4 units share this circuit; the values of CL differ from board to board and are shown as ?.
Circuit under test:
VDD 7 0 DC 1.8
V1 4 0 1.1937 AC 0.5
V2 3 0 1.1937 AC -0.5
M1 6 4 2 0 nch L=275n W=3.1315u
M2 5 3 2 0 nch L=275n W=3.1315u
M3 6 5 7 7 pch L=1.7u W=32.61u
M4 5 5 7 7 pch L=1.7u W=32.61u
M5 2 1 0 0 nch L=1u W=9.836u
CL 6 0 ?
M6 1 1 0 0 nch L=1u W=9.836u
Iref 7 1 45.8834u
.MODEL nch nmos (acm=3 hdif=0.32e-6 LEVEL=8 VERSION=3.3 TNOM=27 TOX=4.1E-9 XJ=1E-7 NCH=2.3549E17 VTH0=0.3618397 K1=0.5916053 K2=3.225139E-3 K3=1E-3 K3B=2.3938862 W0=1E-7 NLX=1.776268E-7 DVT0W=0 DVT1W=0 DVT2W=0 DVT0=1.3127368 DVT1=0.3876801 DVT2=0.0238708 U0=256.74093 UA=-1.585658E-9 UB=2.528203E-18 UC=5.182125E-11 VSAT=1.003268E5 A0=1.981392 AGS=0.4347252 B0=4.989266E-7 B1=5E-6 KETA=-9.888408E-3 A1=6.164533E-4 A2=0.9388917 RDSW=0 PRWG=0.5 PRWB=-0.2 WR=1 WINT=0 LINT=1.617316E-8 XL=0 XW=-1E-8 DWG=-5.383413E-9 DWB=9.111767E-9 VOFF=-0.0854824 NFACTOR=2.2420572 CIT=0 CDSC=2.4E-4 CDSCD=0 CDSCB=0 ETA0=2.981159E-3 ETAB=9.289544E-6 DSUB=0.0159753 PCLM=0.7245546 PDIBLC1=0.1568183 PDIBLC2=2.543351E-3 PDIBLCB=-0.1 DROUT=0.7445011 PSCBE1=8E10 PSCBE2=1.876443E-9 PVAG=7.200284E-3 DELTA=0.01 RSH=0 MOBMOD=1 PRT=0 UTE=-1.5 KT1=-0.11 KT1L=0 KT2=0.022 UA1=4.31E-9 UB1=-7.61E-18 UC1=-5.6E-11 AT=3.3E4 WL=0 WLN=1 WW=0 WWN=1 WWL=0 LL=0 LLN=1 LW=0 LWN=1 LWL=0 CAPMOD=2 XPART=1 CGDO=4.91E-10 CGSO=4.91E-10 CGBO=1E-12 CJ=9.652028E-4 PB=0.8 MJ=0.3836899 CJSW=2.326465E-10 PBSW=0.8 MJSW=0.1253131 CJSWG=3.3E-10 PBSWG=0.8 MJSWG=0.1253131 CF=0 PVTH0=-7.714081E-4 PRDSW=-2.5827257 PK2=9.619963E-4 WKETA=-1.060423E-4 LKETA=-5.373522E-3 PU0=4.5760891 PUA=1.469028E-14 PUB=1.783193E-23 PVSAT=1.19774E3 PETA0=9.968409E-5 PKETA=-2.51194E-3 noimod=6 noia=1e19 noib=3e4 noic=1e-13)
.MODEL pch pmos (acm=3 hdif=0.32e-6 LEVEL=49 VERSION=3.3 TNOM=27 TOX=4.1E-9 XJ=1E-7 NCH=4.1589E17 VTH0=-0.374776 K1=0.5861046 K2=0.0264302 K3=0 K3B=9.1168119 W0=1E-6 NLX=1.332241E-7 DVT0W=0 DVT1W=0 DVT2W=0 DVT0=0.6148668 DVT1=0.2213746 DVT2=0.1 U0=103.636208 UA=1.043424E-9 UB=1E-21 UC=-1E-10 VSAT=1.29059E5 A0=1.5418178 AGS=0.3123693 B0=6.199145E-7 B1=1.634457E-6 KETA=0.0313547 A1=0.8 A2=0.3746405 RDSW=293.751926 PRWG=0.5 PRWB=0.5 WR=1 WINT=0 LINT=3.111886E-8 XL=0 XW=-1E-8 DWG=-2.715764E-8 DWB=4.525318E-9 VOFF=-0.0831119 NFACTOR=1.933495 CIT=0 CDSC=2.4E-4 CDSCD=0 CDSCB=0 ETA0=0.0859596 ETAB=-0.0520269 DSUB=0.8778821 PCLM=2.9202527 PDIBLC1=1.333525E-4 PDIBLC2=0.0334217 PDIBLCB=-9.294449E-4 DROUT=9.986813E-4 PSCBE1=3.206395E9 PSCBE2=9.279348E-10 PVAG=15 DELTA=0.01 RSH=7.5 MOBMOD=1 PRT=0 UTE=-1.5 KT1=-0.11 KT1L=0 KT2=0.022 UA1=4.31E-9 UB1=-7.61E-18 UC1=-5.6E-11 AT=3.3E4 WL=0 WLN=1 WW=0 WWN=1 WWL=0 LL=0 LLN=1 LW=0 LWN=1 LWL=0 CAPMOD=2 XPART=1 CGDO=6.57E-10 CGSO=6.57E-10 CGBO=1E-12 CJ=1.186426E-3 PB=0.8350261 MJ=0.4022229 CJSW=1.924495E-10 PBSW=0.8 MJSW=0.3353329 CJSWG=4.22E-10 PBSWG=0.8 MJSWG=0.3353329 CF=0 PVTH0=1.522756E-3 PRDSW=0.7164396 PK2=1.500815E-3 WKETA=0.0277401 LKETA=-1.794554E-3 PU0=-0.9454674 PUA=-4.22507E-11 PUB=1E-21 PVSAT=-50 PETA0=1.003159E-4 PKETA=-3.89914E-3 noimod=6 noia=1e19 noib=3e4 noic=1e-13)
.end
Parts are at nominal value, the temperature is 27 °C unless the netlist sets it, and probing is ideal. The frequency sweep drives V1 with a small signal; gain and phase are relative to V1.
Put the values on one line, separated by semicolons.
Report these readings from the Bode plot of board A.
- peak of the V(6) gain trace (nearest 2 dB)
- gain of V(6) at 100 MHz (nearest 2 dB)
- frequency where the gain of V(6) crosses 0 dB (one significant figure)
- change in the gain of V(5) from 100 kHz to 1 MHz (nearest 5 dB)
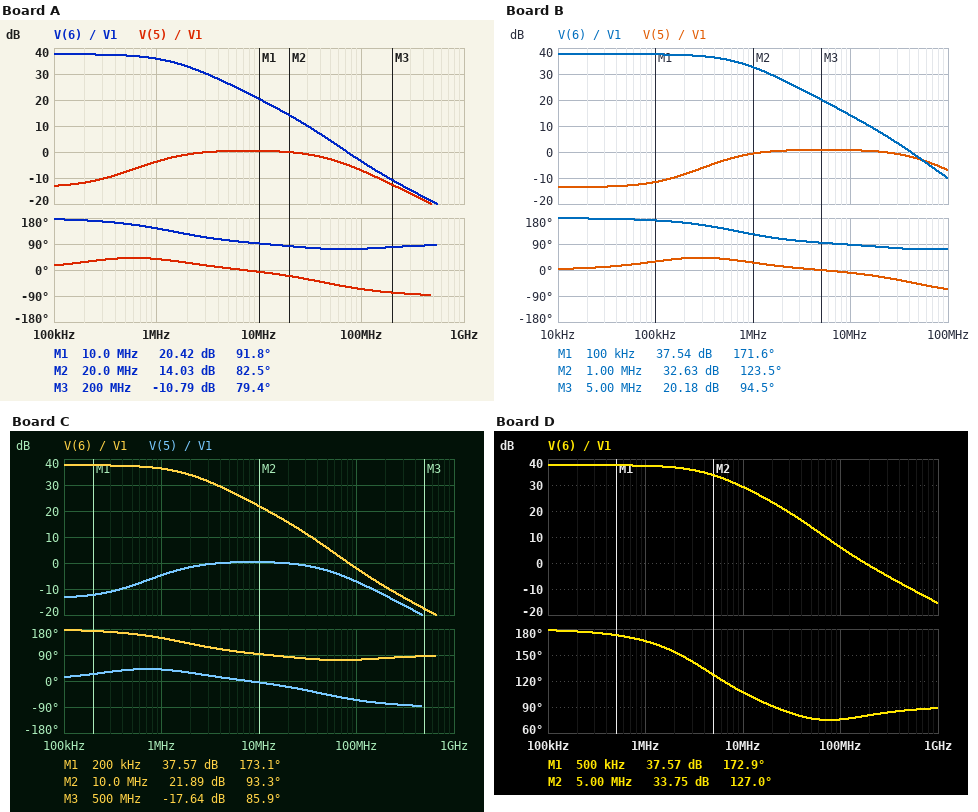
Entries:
38 dB; -4 dB; 70 MHz; 10 dB
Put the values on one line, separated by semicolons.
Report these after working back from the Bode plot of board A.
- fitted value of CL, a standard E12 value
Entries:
680 fF
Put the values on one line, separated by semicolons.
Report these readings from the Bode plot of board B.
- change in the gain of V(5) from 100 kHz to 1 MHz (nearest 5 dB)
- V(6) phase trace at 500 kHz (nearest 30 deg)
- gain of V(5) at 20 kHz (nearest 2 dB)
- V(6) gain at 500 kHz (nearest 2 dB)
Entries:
10 dB; 150 deg; -14 dB; 36 dB
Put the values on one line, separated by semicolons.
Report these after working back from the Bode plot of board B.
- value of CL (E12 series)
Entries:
1.5 pF
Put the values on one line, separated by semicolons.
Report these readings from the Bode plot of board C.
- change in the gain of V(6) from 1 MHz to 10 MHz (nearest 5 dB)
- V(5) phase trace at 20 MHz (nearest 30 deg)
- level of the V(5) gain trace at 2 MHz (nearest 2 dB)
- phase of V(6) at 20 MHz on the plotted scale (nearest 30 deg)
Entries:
-15 dB; -30 deg; -2 dB; 90 deg
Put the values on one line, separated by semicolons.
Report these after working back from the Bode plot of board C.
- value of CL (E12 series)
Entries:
560 fF
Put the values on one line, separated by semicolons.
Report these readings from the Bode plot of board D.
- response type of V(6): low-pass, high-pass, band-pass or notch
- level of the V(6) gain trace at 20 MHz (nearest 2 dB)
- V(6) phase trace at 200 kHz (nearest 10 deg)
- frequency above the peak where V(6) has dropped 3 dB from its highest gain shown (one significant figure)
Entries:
low-pass; 24 dB; 180 deg; 4 MHz
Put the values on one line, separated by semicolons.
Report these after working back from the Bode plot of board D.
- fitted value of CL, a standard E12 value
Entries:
180 fF
